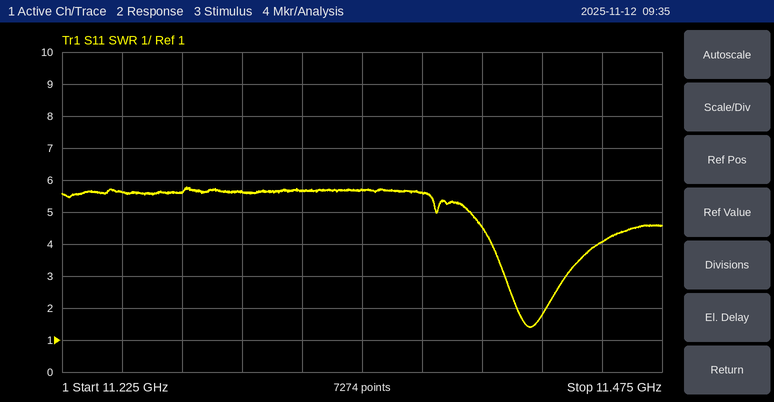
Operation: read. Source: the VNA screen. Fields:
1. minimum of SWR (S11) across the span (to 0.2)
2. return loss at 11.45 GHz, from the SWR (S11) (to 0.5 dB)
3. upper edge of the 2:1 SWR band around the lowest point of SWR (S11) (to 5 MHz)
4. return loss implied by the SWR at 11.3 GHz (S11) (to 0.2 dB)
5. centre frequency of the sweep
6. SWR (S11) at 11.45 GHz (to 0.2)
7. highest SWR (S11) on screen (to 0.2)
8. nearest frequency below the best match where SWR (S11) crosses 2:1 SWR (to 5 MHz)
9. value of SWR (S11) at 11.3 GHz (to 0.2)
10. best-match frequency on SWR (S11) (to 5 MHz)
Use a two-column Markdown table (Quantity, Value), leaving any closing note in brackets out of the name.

| Quantity | Value |
|---|---|
| minimum of SWR (S11) across the span | 1.4 |
| return loss at 11.45 GHz, from the SWR (S11) | 4.5 dB |
| upper edge of the 2:1 SWR band around the lowest point of SWR (S11) | 11.425 GHz |
| return loss implied by the SWR at 11.3 GHz (S11) | 3.2 dB |
| centre frequency of the sweep | 11.35 GHz |
| SWR (S11) at 11.45 GHz | 4.0 |
| highest SWR (S11) on screen | 5.8 |
| nearest frequency below the best match where SWR (S11) crosses 2:1 SWR | 11.415 GHz |
| value of SWR (S11) at 11.3 GHz | 5.6 |
| best-match frequency on SWR (S11) | 11.420 GHz |
